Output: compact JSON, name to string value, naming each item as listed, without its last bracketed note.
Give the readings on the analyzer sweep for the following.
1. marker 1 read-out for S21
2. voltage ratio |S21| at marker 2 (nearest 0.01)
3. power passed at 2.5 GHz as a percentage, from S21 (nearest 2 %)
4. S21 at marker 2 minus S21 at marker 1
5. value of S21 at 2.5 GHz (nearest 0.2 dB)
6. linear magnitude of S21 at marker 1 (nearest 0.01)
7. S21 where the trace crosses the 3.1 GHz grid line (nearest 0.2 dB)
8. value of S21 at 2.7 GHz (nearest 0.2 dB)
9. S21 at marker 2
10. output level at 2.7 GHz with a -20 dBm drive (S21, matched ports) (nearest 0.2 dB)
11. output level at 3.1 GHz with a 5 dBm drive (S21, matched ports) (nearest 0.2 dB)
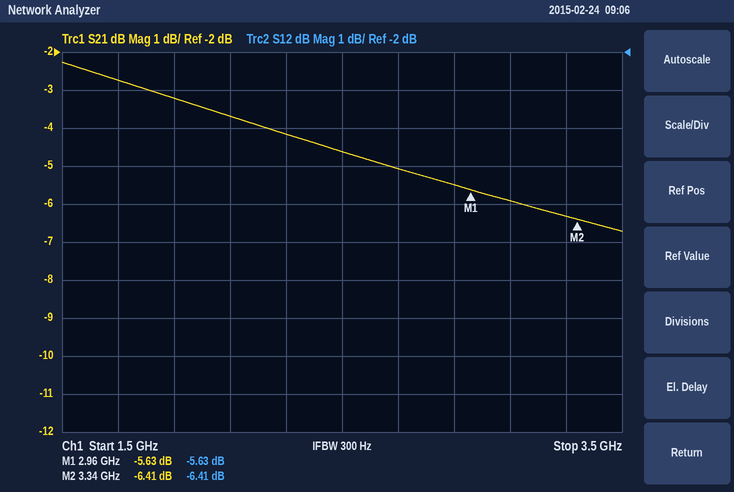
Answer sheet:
{"marker 1 read-out for S21": "-5.63 dB", "voltage ratio |S21| at marker 2": "0.48", "power passed at 2.5 GHz as a percentage, from S21": "34 %", "S21 at marker 2 minus S21 at marker 1": "-0.78 dB", "value of S21 at 2.5 GHz": "-4.6 dB", "linear magnitude of S21 at marker 1": "0.52", "S21 where the trace crosses the 3.1 GHz grid line": "-6.0 dB", "value of S21 at 2.7 GHz": "-5.0 dB", "S21 at marker 2": "-6.41 dB", "output level at 2.7 GHz with a -20 dBm drive (S21, matched ports)": "-25.0 dBm", "output level at 3.1 GHz with a 5 dBm drive (S21, matched ports)": "-1.0 dBm"}
